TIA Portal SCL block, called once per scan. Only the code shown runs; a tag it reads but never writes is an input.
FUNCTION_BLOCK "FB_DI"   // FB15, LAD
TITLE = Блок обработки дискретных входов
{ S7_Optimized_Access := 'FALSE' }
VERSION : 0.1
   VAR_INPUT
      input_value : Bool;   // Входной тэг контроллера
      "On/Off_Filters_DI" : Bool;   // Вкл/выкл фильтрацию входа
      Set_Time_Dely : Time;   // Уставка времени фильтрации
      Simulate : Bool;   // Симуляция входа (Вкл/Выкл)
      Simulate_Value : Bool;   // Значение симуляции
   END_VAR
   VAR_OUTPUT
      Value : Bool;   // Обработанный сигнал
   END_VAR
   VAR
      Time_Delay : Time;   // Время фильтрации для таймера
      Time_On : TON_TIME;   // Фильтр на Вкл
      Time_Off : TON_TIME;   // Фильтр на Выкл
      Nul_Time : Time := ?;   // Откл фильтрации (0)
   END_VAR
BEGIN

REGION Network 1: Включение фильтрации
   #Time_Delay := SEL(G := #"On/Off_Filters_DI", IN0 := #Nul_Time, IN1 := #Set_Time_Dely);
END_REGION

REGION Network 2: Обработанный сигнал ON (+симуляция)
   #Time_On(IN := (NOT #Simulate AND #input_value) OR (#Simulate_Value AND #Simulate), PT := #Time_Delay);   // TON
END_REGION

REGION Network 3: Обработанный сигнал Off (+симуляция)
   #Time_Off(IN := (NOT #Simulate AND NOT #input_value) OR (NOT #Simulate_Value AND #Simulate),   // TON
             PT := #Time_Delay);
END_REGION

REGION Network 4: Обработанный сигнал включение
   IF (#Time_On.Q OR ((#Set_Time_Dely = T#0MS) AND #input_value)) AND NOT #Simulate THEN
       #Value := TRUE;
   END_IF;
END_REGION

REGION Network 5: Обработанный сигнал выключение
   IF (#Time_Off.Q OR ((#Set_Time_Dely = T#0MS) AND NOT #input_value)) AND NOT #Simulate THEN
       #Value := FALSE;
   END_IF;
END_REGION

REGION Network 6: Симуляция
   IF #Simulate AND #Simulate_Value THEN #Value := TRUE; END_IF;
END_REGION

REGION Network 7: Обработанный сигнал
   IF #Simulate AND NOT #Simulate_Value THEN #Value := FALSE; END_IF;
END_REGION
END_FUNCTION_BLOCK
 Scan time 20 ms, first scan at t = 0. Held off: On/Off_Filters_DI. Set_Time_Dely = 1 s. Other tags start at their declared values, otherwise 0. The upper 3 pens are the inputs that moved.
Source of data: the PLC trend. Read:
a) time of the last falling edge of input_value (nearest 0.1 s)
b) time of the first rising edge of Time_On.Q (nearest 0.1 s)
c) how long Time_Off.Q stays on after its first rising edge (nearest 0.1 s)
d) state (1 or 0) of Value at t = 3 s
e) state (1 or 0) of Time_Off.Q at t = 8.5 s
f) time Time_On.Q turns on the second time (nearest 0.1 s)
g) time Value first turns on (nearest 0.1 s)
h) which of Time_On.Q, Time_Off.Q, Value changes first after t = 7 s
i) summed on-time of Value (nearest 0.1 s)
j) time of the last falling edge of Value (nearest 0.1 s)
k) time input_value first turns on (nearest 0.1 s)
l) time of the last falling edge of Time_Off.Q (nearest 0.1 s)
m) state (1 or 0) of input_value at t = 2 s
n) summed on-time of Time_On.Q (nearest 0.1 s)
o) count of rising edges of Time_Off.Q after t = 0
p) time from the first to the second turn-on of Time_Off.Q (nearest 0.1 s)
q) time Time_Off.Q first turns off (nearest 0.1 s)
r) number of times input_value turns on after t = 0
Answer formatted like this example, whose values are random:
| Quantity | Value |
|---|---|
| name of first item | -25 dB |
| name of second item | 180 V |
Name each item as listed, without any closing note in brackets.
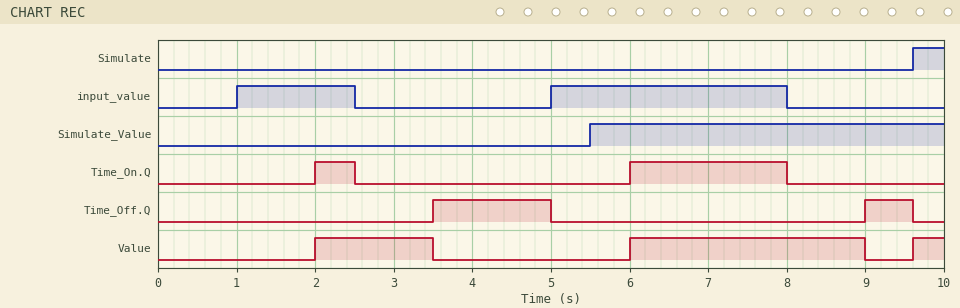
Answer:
| Quantity | Value |
|---|---|
| time of the last falling edge of input_value | 8.0 s |
| time of the first rising edge of Time_On.Q | 2.0 s |
| how long Time_Off.Q stays on after its first rising edge | 1.5 s |
| state (1 or 0) of Value at t = 3 s | 1 |
| state (1 or 0) of Time_Off.Q at t = 8.5 s | 0 |
| time Time_On.Q turns on the second time | 6.0 s |
| time Value first turns on | 2.0 s |
| which of Time_On.Q, Time_Off.Q, Value changes first after t = 7 s | Time_On.Q |
| summed on-time of Value | 4.9 s |
| time of the last falling edge of Value | 9.0 s |
| time input_value first turns on | 1.0 s |
| time of the last falling edge of Time_Off.Q | 9.6 s |
| state (1 or 0) of input_value at t = 2 s | 1 |
| summed on-time of Time_On.Q | 2.5 s |
| count of rising edges of Time_Off.Q after t = 0 | 2 |
| time from the first to the second turn-on of Time_Off.Q | 5.5 s |
| time Time_Off.Q first turns off | 5.0 s |
| number of times input_value turns on after t = 0 | 2 |
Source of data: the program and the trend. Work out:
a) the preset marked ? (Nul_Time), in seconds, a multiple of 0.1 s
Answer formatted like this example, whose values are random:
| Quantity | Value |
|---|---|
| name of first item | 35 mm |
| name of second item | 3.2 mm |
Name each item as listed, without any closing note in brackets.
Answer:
| Quantity | Value |
|---|---|
| the preset marked ? (Nul_Time), in seconds, a multiple of 0.1 s | 1.0 s |
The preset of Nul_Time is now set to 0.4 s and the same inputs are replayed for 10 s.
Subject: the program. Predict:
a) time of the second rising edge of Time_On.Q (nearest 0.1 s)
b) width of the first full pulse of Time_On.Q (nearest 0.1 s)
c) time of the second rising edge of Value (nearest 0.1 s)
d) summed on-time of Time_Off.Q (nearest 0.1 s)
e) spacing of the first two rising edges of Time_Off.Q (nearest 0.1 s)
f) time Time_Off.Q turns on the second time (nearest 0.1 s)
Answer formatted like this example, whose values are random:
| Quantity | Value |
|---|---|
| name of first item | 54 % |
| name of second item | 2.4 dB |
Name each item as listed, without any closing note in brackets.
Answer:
| Quantity | Value |
|---|---|
| time of the second rising edge of Time_On.Q | 5.4 s |
| width of the first full pulse of Time_On.Q | 1.1 s |
| time of the second rising edge of Value | 5.4 s |
| summed on-time of Time_Off.Q | 3.9 s |
| spacing of the first two rising edges of Time_Off.Q | 2.5 s |
| time Time_Off.Q turns on the second time | 2.9 s |
